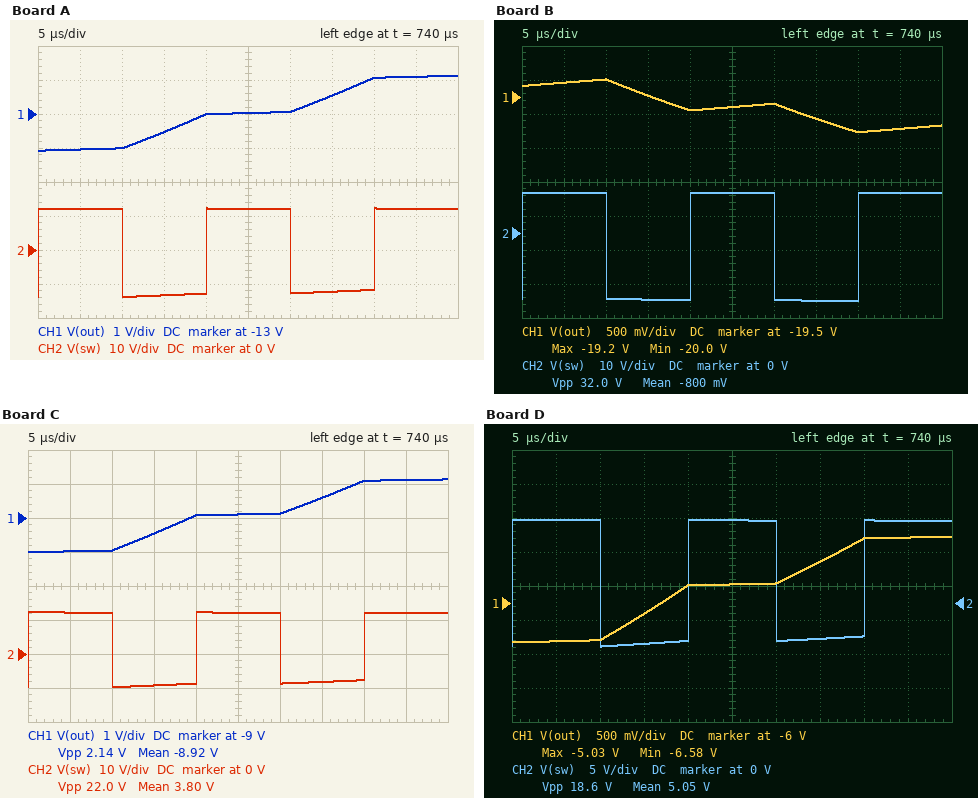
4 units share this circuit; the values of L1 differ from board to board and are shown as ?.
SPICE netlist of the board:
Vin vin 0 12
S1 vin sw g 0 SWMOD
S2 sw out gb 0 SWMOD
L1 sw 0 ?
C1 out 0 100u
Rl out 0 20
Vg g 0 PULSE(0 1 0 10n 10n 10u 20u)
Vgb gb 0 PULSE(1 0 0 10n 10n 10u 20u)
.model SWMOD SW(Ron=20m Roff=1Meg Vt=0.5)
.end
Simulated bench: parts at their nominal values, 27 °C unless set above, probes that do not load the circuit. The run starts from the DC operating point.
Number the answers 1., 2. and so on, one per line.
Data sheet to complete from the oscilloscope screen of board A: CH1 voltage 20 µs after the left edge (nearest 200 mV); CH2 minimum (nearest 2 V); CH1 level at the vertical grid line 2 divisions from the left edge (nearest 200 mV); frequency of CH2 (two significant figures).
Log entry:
1. -13.0 V
2. -14 V
3. -14.0 V
4. 50 kHz
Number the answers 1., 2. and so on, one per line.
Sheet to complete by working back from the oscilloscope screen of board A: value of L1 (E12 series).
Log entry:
1. 68 µH
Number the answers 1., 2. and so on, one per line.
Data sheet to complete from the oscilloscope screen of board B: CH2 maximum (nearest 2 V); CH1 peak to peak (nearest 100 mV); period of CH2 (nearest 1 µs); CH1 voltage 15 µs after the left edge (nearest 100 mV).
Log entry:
1. 12 V
2. 800 mV
3. 20 µs
4. -19.5 V
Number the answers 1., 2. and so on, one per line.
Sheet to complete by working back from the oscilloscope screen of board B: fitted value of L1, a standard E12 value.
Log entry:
1. 220 µH
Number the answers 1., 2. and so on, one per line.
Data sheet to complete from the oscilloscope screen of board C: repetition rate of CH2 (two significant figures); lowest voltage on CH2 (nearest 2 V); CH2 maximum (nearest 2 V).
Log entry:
1. 50 kHz
2. -10 V
3. 12 V
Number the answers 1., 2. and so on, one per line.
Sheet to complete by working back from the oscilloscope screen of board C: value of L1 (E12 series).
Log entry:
1. 56 µH
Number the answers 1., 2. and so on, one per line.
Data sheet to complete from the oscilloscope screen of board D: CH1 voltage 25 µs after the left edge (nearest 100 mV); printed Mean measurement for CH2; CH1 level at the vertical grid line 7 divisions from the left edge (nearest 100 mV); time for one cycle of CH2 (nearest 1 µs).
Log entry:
1. -5.7 V
2. 5.05 V
3. -5.4 V
4. 20 µs
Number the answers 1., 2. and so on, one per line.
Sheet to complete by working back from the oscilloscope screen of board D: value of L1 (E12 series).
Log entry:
1. 47 µH
